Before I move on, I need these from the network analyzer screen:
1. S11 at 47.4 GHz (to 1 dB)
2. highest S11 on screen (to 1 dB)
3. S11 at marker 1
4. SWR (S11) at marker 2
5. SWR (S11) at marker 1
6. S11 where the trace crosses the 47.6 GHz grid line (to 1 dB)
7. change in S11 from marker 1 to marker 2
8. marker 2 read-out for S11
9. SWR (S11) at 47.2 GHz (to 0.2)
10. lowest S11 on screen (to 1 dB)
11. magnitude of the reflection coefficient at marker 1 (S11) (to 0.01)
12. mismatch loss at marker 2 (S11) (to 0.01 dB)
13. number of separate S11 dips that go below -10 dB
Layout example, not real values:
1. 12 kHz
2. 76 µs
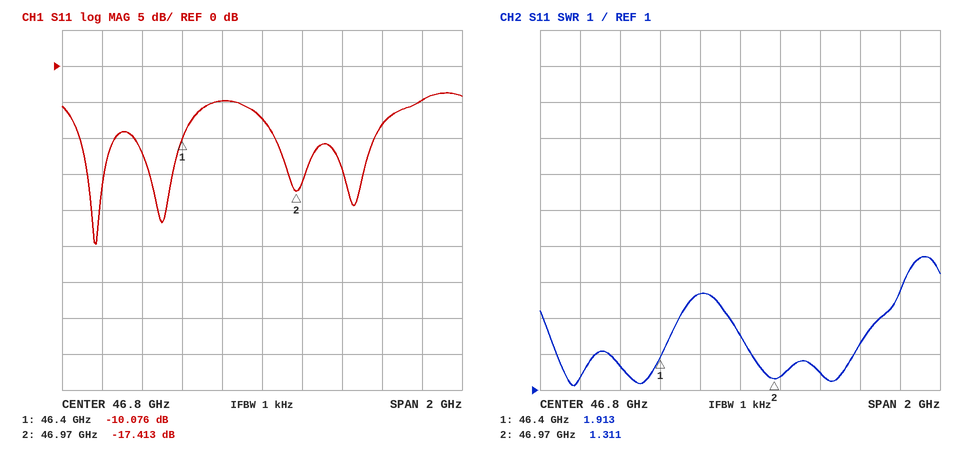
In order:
1. -8 dB
2. -4 dB
3. -10.076 dB
4. 1.311
5. 1.913
6. -5 dB
7. -7.337 dB
8. -17.413 dB
9. 1.4
10. -25 dB
11. 0.31
12. 0.08 dB
13. 4
